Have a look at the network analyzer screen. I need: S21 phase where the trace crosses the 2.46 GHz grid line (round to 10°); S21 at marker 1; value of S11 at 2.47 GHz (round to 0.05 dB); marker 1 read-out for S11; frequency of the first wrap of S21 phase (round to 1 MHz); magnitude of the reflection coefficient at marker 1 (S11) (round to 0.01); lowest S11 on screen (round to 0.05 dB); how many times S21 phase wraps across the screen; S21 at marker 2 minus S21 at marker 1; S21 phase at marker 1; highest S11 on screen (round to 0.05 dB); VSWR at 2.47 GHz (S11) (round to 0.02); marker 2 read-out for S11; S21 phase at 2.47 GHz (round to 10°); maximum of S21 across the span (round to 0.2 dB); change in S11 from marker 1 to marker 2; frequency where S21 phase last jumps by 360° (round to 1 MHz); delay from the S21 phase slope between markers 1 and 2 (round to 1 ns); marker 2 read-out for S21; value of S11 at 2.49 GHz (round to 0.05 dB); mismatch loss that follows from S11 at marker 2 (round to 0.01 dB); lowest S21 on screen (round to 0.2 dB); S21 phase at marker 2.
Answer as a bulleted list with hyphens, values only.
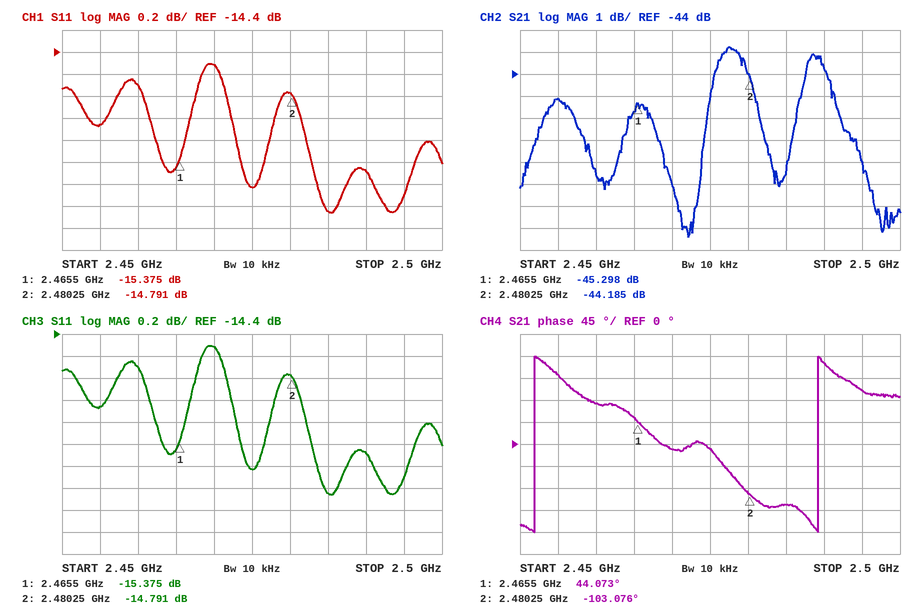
- 80°
- -45.298 dB
- -14.50 dB
- -15.375 dB
- 2.452 GHz
- 0.17
- -15.85 dB
- 2
- 1.113 dB
- 44.073°
- -14.50 dB
- 1.46
- -14.791 dB
- -10°
- -42.8 dB
- 0.584 dB
- 2.489 GHz
- 28 ns
- -44.185 dB
- -15.50 dB
- 0.15 dB
- -51.4 dB
- -103.076°
